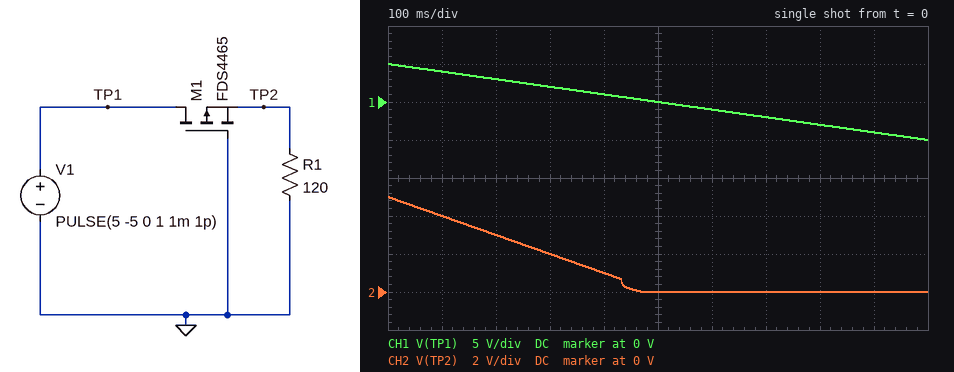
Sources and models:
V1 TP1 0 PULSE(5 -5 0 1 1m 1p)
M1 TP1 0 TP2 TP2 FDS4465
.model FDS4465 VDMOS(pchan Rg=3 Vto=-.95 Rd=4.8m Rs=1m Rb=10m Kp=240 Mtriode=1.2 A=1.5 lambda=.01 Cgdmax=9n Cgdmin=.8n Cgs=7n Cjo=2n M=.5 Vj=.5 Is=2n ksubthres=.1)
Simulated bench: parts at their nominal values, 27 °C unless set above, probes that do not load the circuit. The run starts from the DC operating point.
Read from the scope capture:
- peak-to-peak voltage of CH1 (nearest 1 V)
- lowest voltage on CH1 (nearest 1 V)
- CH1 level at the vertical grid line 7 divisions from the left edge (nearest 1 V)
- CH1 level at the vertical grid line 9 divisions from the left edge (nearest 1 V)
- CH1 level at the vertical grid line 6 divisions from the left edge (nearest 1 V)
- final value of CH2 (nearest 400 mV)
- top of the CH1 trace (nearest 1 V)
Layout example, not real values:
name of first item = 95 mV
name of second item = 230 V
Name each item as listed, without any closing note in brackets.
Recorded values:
peak-to-peak voltage of CH1 = 10 V
lowest voltage on CH1 = -5 V
CH1 level at the vertical grid line 7 divisions from the left edge = -2 V
CH1 level at the vertical grid line 9 divisions from the left edge = -4 V
CH1 level at the vertical grid line 6 divisions from the left edge = -1 V
final value of CH2 = 0 V
top of the CH1 trace = 5 V
